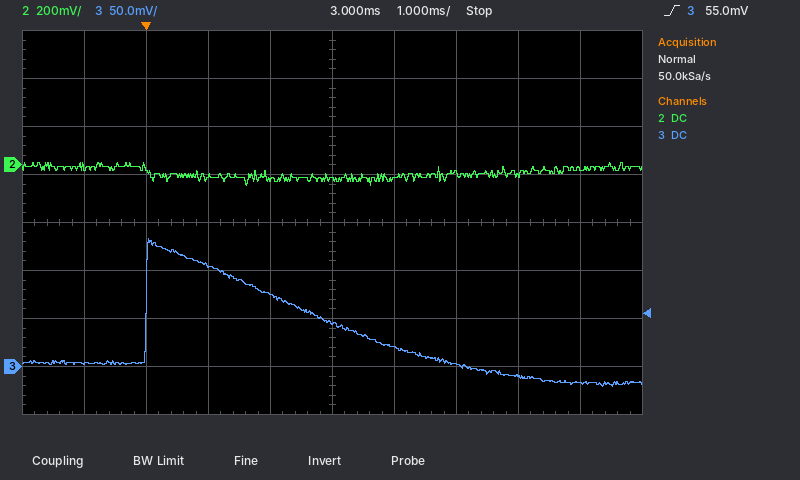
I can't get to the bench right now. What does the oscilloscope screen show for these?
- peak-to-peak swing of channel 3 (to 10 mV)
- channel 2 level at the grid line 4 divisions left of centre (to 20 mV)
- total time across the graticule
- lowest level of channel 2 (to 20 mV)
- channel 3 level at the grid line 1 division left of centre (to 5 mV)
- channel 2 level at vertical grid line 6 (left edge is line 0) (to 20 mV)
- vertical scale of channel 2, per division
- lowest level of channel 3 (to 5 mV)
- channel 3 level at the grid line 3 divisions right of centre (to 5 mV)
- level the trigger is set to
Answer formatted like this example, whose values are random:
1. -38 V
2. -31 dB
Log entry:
1. 150 mV
2. 0 mV
3. 10 ms
4. -80 mV
5. 75 mV
6. -60 mV
7. 200 mV
8. -20 mV
9. -10 mV
10. 55.0 mV
